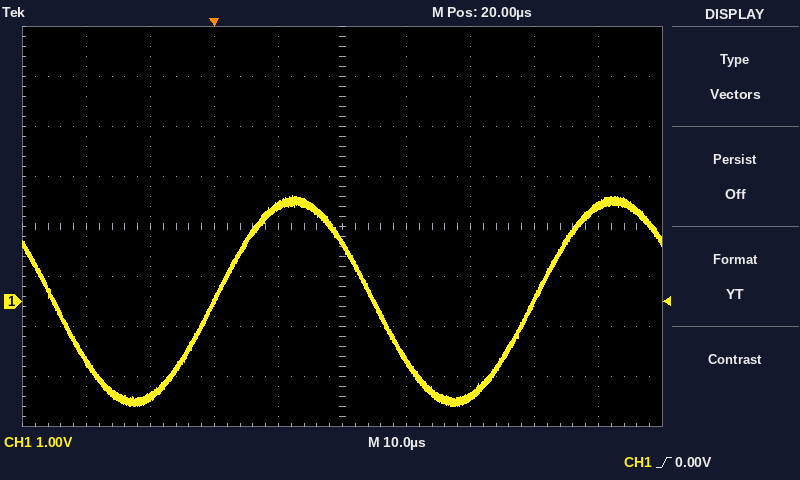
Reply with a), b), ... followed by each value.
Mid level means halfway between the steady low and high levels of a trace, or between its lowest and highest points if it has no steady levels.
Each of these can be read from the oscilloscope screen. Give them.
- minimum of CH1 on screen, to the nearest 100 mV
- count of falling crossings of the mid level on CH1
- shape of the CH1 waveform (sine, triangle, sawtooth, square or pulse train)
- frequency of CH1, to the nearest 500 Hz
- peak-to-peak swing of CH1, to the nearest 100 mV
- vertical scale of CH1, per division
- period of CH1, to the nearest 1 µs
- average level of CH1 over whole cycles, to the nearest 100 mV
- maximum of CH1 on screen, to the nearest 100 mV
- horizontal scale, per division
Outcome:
a) -2.1 V
b) 2
c) sine
d) 20.0 kHz
e) 4.2 V
f) 1 V
g) 50 µs
h) 0.0 V
i) 2.1 V
j) 10 µs
